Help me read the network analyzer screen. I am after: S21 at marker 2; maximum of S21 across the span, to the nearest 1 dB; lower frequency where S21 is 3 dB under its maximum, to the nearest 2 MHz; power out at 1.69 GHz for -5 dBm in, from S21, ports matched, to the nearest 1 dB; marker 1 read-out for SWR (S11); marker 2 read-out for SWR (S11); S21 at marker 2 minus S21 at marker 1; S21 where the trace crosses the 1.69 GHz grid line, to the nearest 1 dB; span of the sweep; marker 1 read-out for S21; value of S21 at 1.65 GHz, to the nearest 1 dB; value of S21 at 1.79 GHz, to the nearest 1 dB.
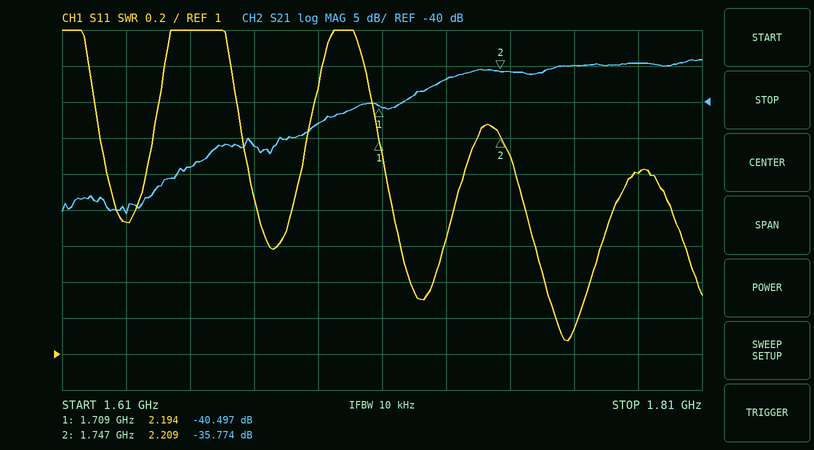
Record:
-35.774 dB
-34 dB
1.728 GHz
-48 dBm
2.194
2.209
4.723 dB
-43 dB
200 MHz
-40.497 dB
-49 dB
-35 dB
